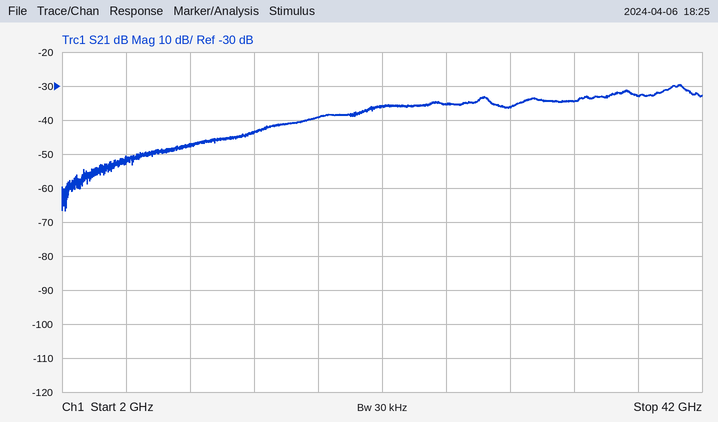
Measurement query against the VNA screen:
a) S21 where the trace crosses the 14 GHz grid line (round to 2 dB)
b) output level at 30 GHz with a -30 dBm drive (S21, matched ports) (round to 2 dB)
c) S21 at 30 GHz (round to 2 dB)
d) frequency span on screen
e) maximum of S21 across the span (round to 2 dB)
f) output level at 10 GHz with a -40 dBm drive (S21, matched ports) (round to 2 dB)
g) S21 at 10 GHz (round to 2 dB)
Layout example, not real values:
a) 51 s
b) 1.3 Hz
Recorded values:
a) -44 dB
b) -66 dBm
c) -36 dB
d) 40 GHz
e) -30 dB
f) -88 dBm
g) -48 dB
